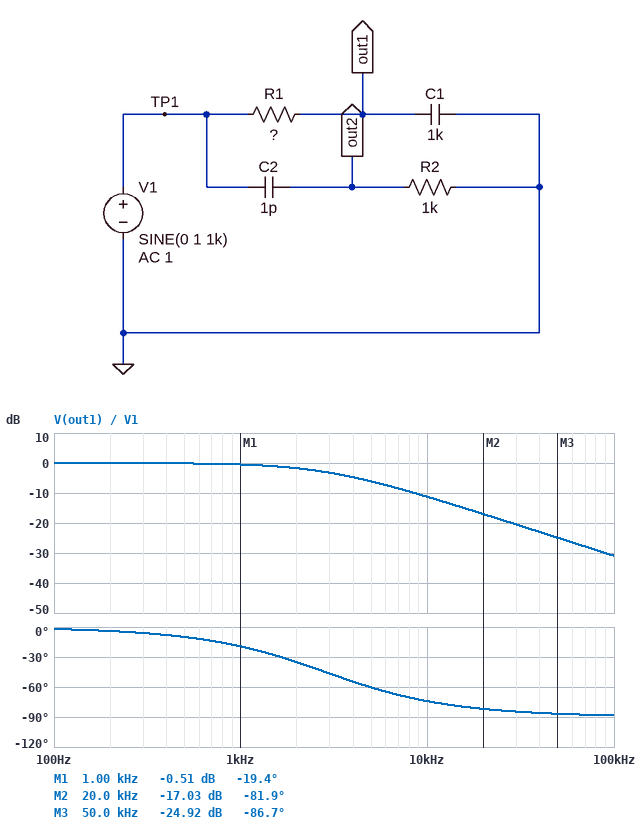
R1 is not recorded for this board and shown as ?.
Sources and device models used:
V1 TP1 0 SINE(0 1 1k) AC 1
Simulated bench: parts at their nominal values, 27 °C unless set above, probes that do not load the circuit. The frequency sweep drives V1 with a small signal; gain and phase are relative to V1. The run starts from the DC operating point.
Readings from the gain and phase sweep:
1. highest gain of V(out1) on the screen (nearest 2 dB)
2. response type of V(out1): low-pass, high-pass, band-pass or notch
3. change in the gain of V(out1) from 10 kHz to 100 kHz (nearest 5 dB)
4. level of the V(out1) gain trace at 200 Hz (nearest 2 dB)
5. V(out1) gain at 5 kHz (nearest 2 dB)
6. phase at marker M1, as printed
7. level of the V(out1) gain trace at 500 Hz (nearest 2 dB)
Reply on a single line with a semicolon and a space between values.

0 dB; low-pass; -20 dB; 0 dB; -6 dB; -19.4 deg; 0 dB
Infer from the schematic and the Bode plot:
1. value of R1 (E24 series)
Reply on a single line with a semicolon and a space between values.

56 nΩ
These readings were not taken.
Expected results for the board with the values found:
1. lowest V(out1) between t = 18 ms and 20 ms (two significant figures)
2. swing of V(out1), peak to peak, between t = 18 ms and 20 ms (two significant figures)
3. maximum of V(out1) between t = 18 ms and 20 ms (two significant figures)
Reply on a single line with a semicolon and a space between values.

-940 mV; 1.9 V; 940 mV
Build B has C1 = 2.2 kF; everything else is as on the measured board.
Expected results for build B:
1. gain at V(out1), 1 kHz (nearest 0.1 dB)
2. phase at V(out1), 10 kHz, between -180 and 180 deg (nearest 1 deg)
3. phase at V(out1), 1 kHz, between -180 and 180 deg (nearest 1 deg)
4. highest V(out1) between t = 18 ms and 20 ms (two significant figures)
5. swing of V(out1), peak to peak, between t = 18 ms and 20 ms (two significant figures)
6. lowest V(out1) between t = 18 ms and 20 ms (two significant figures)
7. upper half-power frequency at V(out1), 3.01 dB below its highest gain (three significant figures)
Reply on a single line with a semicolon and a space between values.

-2.0 dB; -83 deg; -38 deg; 790 mV; 1.6 V; -790 mV; 1.29 kHz
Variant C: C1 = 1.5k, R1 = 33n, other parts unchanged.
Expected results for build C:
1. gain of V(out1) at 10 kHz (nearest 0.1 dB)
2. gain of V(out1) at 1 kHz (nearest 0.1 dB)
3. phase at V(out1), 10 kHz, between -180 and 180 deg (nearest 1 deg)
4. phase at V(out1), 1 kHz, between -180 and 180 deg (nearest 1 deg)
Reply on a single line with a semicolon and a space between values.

-10.3 dB; -0.4 dB; -72 deg; -17 deg
